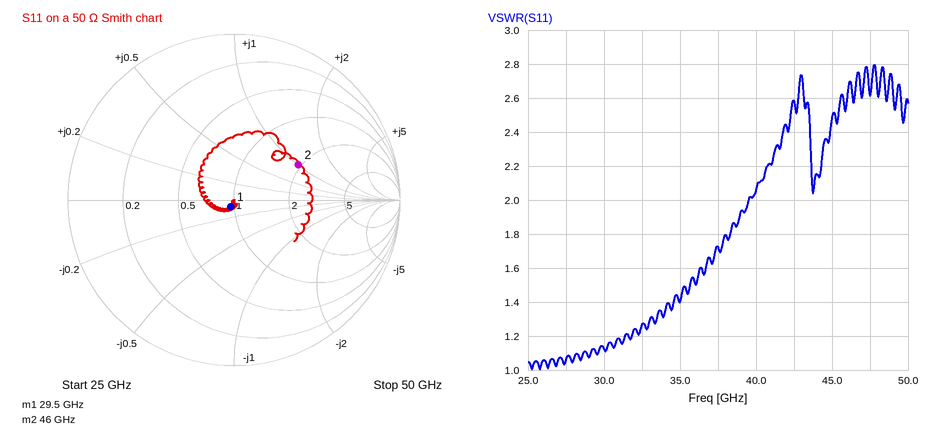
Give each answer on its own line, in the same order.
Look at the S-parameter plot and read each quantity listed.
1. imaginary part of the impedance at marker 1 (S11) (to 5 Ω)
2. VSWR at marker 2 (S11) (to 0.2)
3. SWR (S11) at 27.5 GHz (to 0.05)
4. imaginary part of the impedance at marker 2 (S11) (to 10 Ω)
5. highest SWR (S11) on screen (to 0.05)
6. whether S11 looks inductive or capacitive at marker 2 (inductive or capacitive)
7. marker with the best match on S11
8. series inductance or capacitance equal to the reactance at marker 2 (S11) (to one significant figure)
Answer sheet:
-5 Ω
2.6
1.05
+50 Ω
2.80
inductive
marker 1
200 pH
